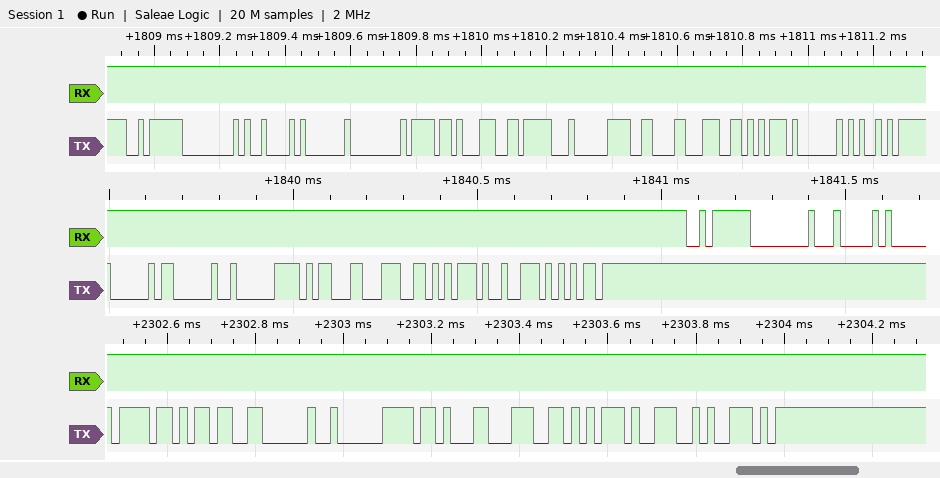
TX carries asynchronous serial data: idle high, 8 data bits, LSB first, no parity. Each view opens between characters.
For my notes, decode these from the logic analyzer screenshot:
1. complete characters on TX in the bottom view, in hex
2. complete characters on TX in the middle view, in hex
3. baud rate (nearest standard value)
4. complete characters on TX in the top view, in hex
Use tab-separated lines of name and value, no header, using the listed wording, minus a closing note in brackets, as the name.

complete characters on TX in the bottom view, in hex	6F, 9B, 20, E0, 8B, 9C, 75, 4E, AE
complete characters on TX in the middle view, in hex	A0, 20, E0, 8D, 9C, 75, 72, B5
baud rate	57600 baud
complete characters on TX in the top view, in hex	FA, 00, 09, 01, 00, 6F, 9C, 1F, E0, 86, 9C, 75, 40, A9
